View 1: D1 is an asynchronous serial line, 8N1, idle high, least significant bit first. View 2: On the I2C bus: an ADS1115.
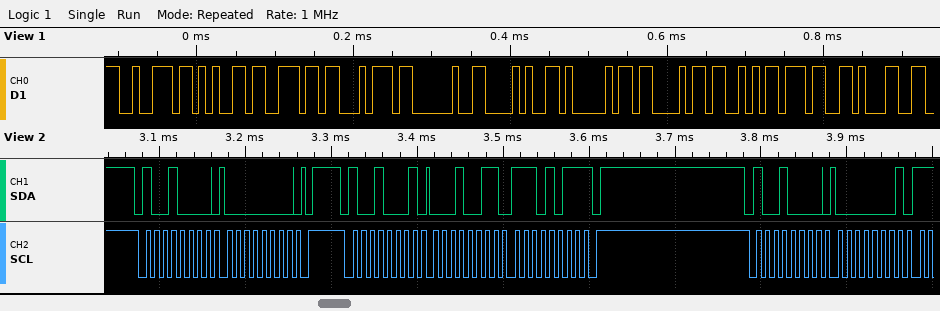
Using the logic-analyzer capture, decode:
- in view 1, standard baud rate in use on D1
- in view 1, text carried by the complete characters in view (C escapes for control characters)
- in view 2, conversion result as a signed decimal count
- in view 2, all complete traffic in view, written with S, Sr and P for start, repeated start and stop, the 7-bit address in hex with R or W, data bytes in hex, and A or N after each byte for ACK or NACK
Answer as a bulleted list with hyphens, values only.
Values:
- 115200 baud
- "rent (ACS71"
- 5099
- S 48W A 00 A P S 48R A 13 A EB N P S 48W A 01 A
